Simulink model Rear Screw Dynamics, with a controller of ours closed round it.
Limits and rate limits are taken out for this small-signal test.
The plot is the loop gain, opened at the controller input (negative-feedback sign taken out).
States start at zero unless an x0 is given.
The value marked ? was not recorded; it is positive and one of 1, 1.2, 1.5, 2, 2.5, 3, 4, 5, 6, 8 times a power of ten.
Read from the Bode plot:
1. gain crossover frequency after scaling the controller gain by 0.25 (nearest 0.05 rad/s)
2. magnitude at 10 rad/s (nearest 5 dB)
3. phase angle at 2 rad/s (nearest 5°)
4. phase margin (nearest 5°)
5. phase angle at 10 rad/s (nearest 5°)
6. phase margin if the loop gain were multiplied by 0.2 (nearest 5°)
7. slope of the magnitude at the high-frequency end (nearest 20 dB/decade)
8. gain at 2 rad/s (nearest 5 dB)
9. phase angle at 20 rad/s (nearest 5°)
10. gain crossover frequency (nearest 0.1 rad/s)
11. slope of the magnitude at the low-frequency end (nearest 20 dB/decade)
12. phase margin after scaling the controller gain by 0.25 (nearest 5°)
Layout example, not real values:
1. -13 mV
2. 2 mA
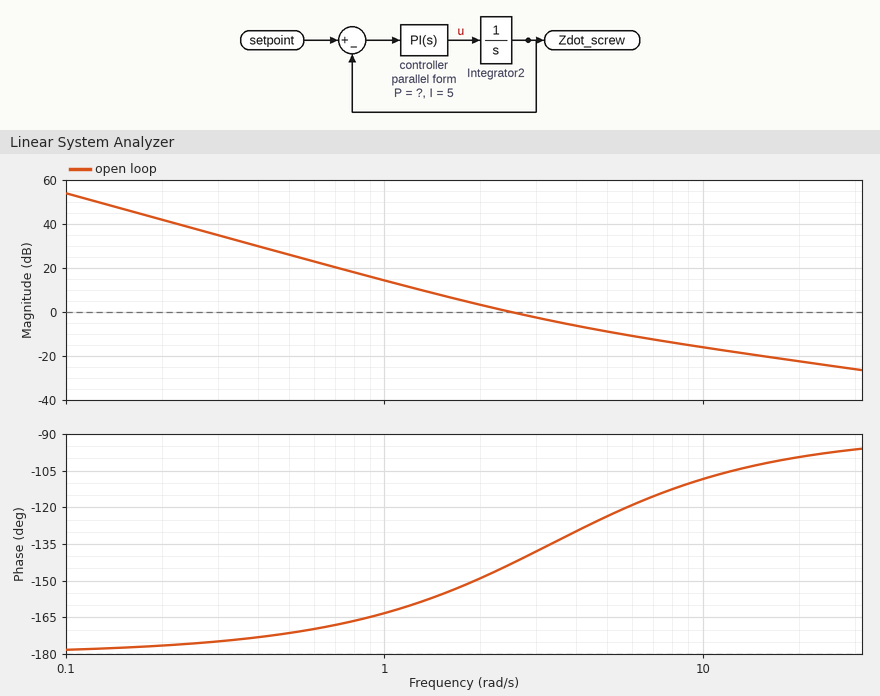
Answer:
1. 1.15 rad/s
2. -15 dB
3. -150°
4. 35°
5. -110°
6. 15°
7. -20 dB/decade
8. 5 dB
9. -100°
10. 2.5 rad/s
11. -40 dB/decade
12. 20°
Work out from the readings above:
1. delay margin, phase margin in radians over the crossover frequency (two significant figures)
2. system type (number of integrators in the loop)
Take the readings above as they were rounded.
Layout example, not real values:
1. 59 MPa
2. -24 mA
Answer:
1. 0.24 s
2. 2
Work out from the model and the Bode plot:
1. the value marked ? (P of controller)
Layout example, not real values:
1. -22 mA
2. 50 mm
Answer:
1. 1.5
